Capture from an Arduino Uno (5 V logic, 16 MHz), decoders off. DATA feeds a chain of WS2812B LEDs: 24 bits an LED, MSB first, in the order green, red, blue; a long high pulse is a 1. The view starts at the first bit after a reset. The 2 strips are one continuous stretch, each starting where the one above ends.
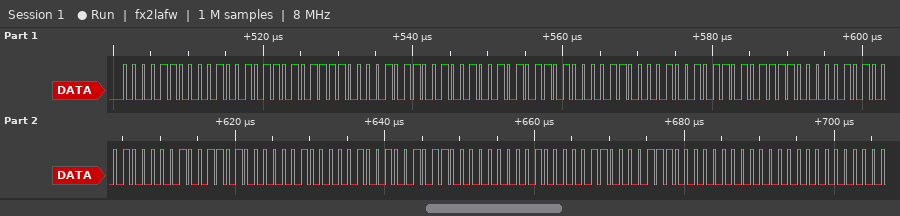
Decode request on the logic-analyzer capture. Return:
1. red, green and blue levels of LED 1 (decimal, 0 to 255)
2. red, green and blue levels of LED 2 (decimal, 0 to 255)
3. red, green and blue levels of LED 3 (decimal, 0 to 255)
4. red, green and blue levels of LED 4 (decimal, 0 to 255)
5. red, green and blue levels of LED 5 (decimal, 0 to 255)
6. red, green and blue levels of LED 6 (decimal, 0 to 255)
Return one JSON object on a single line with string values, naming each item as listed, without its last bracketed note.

{"red, green and blue levels of LED 1": "37, 12, 175", "red, green and blue levels of LED 2": "36, 11, 173", "red, green and blue levels of LED 3": "37, 12, 175", "red, green and blue levels of LED 4": "16, 5, 77", "red, green and blue levels of LED 5": "9, 2, 44", "red, green and blue levels of LED 6": "6, 1, 28"}
